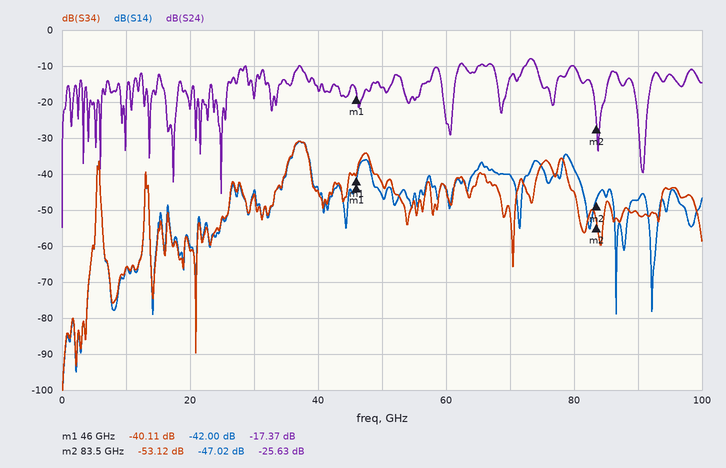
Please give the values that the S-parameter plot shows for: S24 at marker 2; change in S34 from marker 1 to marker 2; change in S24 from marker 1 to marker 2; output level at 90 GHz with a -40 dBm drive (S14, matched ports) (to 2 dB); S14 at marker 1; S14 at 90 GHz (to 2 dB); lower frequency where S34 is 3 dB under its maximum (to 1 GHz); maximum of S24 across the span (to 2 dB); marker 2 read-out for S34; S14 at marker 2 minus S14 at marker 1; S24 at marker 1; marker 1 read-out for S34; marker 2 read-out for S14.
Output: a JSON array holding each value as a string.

["-25.63 dB", "-13.01 dB", "-8.26 dB", "-88 dBm", "-42.00 dB", "-48 dB", "36 GHz", "-8 dB", "-53.12 dB", "-5.02 dB", "-17.37 dB", "-40.11 dB", "-47.02 dB"]
